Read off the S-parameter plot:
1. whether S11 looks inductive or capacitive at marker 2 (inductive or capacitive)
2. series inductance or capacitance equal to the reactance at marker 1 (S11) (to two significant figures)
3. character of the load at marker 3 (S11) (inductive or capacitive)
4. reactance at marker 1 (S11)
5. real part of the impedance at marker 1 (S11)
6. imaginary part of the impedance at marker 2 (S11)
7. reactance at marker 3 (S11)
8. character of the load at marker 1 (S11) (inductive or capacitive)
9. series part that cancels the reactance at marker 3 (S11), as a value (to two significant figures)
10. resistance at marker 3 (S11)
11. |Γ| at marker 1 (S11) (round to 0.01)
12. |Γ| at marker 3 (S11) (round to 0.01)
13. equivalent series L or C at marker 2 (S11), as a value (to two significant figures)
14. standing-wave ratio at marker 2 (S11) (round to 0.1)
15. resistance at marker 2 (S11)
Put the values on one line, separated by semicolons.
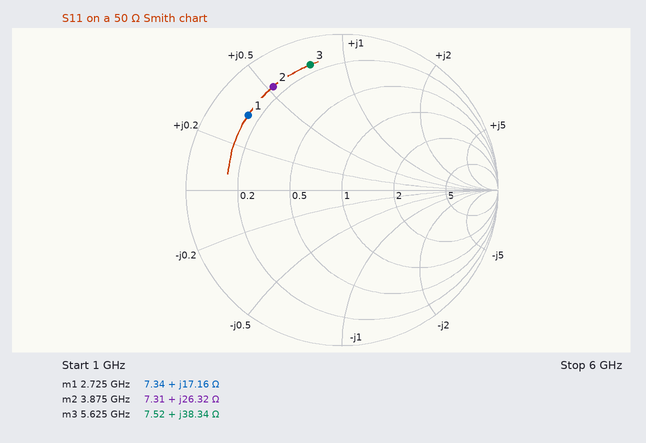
inductive; 1.0 nH; inductive; +17.16 Ω; 7.34 Ω; +26.32 Ω; +38.34 Ω; inductive; 740 fF; 7.52 Ω; 0.77; 0.83; 1.1 nH; 8.8; 7.31 Ω
